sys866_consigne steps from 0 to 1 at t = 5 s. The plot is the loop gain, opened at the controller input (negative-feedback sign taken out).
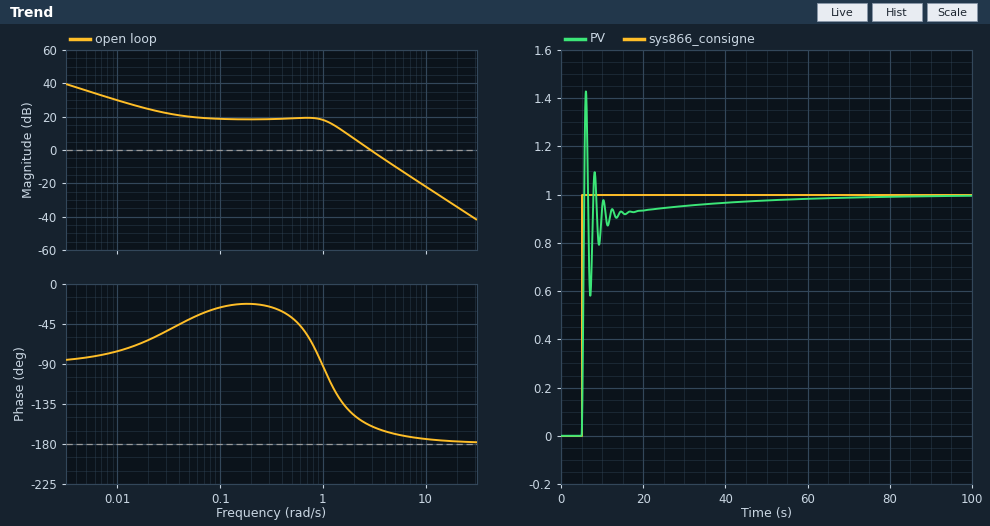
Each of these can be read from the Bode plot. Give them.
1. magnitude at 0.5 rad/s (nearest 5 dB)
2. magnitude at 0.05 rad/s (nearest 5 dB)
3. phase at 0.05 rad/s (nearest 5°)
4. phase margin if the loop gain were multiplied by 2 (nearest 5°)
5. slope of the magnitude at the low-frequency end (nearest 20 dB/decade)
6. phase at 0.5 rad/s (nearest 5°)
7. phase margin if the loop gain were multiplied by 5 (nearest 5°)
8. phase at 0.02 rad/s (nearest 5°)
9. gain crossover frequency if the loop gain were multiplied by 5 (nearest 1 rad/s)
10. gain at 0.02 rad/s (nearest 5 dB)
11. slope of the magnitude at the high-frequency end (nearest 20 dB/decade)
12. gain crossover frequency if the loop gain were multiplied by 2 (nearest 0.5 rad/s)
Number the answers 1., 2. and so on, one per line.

1. 20 dB
2. 20 dB
3. -40°
4. 15°
5. -20 dB/decade
6. -40°
7. 10°
8. -65°
9. 6 rad/s
10. 25 dB
11. -40 dB/decade
12. 4.0 rad/s
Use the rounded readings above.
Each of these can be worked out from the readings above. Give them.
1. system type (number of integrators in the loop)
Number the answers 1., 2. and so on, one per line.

1. 1
